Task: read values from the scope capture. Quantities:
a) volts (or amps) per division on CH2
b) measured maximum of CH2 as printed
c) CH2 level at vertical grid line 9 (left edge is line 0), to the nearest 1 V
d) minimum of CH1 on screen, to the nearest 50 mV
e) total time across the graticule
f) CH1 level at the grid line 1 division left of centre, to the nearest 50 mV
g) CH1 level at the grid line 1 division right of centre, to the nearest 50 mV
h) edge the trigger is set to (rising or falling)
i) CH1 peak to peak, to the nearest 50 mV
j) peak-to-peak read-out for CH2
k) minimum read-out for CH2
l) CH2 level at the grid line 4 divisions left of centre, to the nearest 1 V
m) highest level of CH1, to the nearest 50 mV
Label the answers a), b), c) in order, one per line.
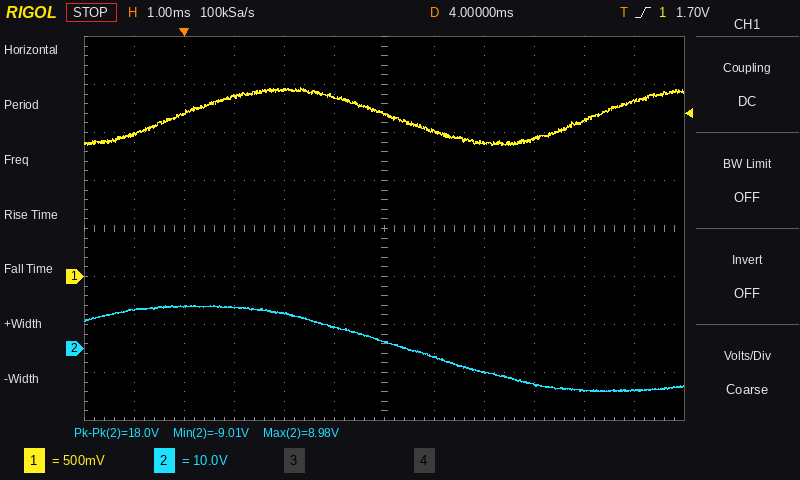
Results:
a) 10 V
b) 8.98 V
c) -8 V
d) 1.35 V
e) 12 ms
f) 1.85 V
g) 1.50 V
h) rising
i) 600 mV
j) 18.0 V
k) -9.01 V
l) 9 V
m) 1.95 V
